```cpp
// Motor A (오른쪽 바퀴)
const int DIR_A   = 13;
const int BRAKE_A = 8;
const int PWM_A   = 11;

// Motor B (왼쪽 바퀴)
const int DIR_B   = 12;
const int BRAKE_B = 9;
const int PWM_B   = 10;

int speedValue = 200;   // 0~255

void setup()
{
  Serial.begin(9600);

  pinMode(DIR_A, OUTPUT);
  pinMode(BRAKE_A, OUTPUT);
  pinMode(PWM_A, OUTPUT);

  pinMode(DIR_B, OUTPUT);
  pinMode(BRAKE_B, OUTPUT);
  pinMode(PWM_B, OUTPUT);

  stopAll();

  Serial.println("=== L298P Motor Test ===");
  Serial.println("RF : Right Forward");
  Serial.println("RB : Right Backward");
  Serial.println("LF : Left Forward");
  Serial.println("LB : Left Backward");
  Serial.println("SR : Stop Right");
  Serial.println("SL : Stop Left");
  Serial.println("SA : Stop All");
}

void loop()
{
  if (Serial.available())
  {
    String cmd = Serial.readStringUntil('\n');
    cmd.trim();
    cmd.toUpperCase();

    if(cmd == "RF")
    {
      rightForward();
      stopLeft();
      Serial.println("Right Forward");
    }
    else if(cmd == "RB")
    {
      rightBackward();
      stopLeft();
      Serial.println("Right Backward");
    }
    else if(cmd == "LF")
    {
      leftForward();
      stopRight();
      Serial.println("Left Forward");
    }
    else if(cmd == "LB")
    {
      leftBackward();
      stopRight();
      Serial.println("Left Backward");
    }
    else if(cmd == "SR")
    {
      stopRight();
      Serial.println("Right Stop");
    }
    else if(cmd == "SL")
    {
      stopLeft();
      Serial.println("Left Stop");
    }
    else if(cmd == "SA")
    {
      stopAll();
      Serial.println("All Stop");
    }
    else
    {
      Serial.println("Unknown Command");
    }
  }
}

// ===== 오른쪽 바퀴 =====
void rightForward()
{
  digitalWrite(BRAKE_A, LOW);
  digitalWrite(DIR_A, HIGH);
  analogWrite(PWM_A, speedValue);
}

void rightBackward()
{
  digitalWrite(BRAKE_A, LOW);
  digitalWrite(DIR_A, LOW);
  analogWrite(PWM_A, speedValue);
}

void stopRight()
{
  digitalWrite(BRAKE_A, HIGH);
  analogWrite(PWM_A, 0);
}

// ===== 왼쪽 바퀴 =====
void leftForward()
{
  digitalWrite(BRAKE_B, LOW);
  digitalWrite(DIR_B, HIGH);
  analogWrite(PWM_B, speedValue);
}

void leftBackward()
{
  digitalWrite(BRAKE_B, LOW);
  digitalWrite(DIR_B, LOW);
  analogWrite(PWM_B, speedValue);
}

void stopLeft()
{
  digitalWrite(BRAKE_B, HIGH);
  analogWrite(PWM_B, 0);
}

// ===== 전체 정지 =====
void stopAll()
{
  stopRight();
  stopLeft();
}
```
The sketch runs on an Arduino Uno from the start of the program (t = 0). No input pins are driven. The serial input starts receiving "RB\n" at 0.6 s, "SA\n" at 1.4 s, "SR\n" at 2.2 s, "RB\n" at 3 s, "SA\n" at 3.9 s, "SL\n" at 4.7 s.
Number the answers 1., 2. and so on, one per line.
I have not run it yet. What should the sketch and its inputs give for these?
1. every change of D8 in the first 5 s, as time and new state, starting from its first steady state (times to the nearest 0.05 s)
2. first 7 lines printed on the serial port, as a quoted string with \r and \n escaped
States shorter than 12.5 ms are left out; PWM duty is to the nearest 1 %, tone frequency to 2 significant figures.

1. 0 s high; 0.6 s low; 1.4 s high; 3 s low; 3.9 s high
2. "=== L298P Motor Test ===\r\nRF : Right Forward\r\nRB : Right Backward\r\nLF : Left Forward\r\nLB : Left Backward\r\nSR : Stop Right\r\nSL : Stop Left\r\n"
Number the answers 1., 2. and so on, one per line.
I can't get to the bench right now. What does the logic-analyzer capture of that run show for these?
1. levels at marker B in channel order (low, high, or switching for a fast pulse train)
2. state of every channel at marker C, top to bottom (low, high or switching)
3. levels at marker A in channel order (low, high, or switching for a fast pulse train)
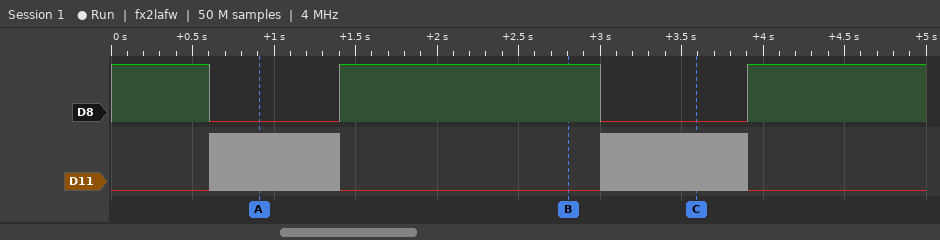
1. D8 high, D11 low
2. D8 low, D11 switching
3. D8 low, D11 switching
